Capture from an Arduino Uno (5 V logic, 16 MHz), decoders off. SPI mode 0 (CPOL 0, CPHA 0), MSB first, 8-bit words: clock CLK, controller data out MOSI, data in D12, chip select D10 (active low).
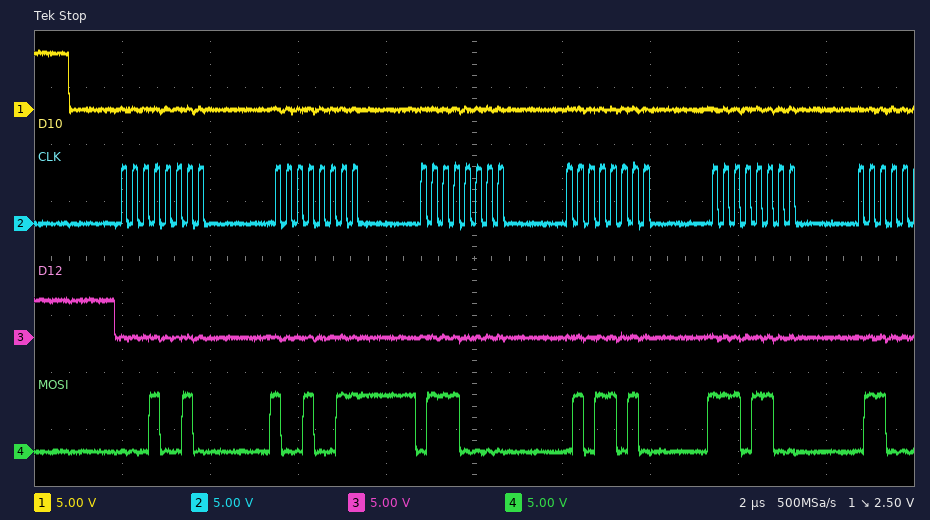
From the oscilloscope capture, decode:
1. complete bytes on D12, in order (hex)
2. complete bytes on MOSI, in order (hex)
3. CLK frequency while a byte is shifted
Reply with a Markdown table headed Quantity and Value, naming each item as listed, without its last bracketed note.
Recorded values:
| Quantity | Value |
|---|---|
| complete bytes on D12, in order | 00 00 00 00 00 |
| complete bytes on MOSI, in order | 12 93 70 5A EC |
| CLK frequency while a byte is shifted | 4 MHz |
